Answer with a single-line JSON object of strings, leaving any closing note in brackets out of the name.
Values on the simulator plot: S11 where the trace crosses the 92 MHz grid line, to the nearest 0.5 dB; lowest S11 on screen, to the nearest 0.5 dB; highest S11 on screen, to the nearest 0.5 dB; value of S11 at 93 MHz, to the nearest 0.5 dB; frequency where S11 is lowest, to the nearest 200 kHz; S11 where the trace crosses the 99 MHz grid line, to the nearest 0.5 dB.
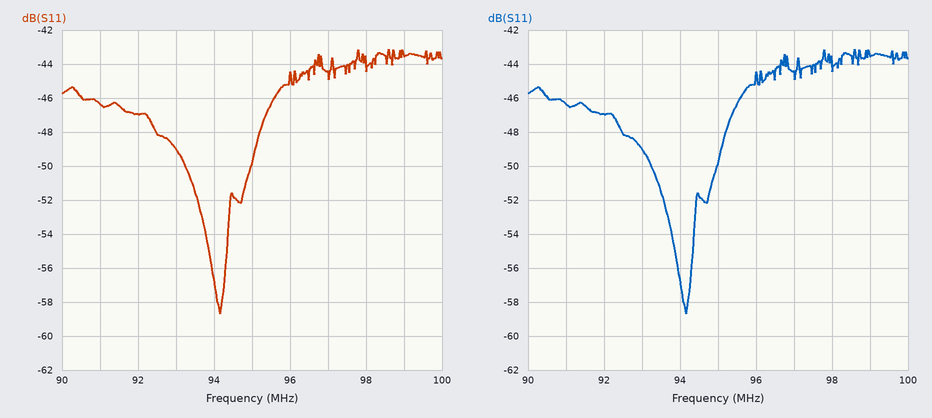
{"S11 where the trace crosses the 92 MHz grid line, to the nearest 0.5 dB": "-47.0 dB", "lowest S11 on screen, to the nearest 0.5 dB": "-58.5 dB", "highest S11 on screen, to the nearest 0.5 dB": "-43.0 dB", "value of S11 at 93 MHz, to the nearest 0.5 dB": "-49.0 dB", "frequency where S11 is lowest, to the nearest 200 kHz": "94.2 MHz", "S11 where the trace crosses the 99 MHz grid line, to the nearest 0.5 dB": "-43.5 dB"}
